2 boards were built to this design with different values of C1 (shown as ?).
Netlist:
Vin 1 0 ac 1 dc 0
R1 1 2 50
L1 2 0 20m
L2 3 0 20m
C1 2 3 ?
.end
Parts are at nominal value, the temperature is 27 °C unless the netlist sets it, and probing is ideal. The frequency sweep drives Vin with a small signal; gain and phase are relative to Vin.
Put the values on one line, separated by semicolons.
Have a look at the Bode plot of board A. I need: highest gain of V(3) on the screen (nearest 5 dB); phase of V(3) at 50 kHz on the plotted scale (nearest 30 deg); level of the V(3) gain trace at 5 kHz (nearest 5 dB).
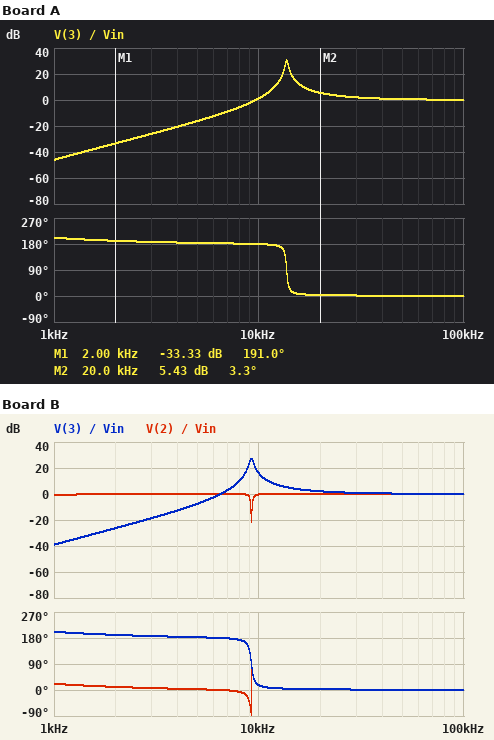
30 dB; 0 deg; -15 dB
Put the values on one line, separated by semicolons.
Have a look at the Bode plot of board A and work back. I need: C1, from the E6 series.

6.8 nF
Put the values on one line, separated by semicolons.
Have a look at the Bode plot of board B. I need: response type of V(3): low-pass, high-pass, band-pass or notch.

high-pass
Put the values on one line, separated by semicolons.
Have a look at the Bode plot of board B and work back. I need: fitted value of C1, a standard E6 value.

15 nF
